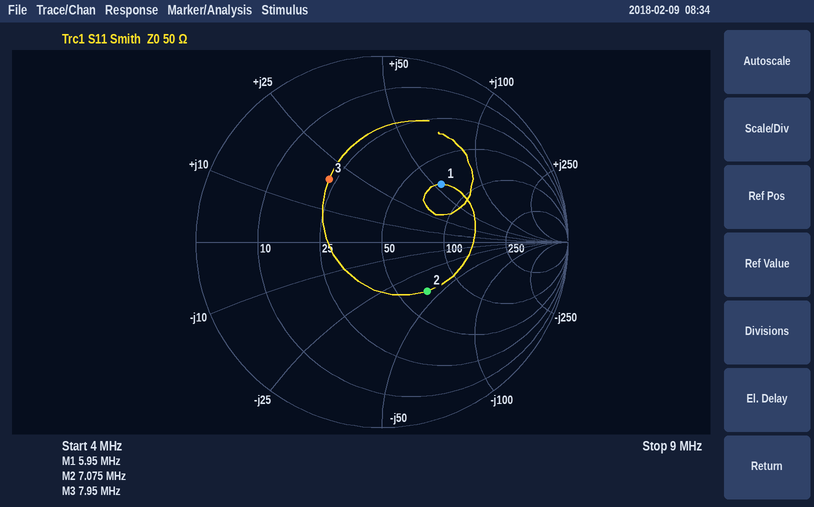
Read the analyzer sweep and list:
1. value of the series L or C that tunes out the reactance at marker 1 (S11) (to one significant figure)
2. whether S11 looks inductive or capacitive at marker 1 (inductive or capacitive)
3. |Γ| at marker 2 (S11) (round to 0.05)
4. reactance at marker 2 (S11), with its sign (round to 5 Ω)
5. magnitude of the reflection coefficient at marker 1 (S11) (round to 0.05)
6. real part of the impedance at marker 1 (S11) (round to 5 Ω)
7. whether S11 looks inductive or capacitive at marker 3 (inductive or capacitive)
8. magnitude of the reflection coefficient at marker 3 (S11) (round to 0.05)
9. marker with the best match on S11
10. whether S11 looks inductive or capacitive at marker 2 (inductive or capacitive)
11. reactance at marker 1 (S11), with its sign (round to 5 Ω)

500 pF
inductive
0.35
-40 Ω
0.45
70 Ω
inductive
0.45
marker 2
capacitive
+55 Ω
